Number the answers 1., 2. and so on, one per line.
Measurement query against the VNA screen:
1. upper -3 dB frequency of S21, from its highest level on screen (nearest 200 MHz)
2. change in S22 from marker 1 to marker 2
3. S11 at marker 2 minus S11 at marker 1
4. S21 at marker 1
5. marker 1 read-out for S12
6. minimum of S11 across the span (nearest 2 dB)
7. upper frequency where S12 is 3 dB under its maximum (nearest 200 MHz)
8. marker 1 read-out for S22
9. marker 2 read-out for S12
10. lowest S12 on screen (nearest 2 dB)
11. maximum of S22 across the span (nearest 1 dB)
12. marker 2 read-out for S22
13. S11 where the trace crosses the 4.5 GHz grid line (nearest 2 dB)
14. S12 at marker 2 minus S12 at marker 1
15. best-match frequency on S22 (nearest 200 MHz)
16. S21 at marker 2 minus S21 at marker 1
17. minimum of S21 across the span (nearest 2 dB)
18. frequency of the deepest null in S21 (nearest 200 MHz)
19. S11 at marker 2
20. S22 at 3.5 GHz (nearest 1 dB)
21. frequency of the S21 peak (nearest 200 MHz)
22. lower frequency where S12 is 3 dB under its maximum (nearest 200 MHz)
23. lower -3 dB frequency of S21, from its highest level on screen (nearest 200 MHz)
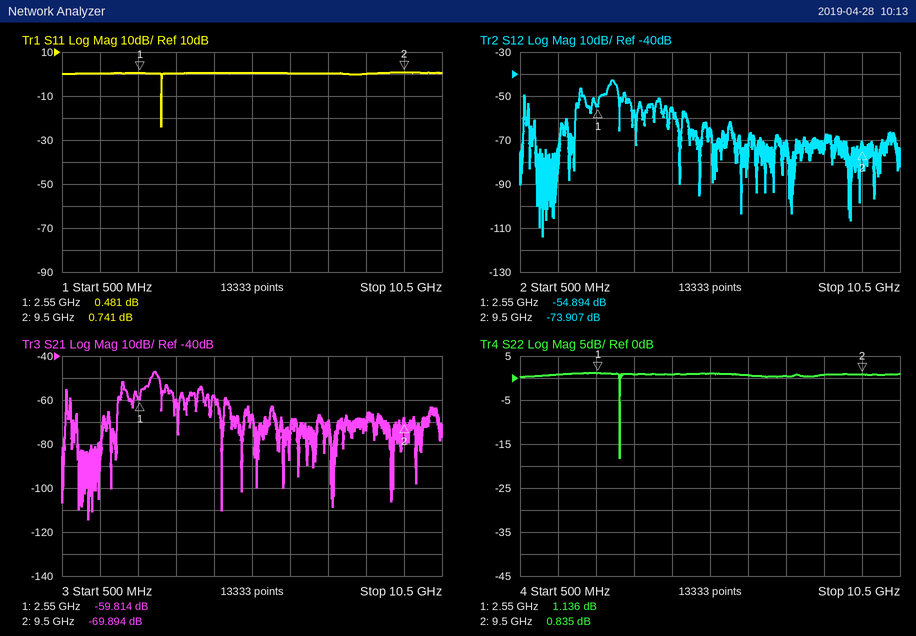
1. 3.0 GHz
2. -0.301 dB
3. 0.260 dB
4. -59.814 dB
5. -54.894 dB
6. -24 dB
7. 3.0 GHz
8. 1.136 dB
9. -73.907 dB
10. -114 dB
11. 1 dB
12. 0.835 dB
13. 0 dB
14. -19.013 dB
15. 3.2 GHz
16. -10.080 dB
17. -114 dB
18. 1.2 GHz
19. 0.741 dB
20. 1 dB
21. 3.0 GHz
22. 2.8 GHz
23. 2.8 GHz
